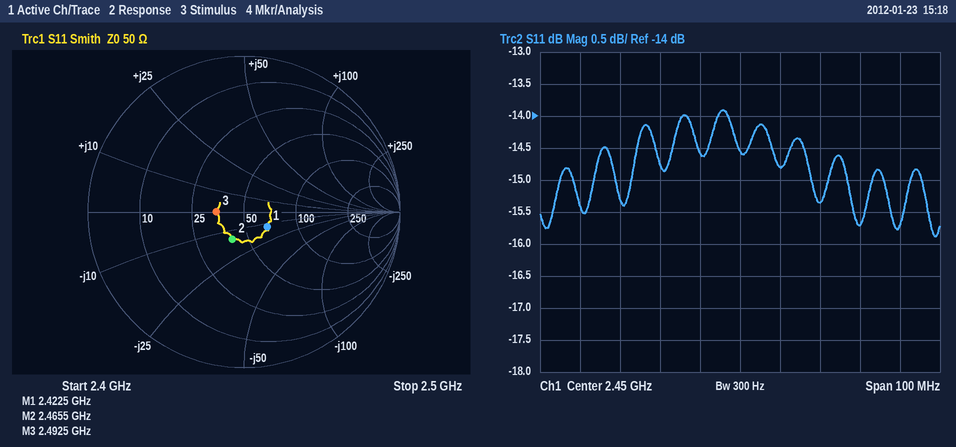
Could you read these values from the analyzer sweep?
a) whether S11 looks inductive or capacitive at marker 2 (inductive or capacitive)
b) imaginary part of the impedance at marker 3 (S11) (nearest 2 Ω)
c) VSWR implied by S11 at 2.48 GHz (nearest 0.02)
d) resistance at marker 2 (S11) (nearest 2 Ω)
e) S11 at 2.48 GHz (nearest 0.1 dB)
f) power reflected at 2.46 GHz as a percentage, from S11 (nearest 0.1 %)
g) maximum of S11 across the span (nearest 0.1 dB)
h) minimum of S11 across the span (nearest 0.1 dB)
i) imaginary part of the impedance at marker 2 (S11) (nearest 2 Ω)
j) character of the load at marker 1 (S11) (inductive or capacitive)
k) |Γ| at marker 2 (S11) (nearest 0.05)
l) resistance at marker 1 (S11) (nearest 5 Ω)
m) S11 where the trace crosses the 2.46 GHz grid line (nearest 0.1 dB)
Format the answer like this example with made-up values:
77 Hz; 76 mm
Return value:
capacitive; 0 Ω; 1.40; 40 Ω; -15.7 dB; 3.3 %; -13.9 dB; -15.9 dB; -14 Ω; capacitive; 0.20; 65 Ω; -14.8 dB
